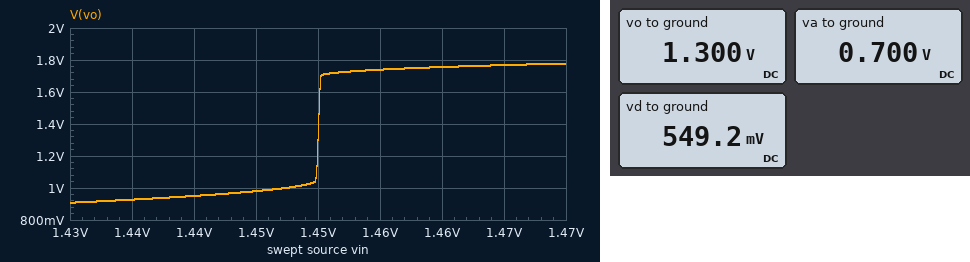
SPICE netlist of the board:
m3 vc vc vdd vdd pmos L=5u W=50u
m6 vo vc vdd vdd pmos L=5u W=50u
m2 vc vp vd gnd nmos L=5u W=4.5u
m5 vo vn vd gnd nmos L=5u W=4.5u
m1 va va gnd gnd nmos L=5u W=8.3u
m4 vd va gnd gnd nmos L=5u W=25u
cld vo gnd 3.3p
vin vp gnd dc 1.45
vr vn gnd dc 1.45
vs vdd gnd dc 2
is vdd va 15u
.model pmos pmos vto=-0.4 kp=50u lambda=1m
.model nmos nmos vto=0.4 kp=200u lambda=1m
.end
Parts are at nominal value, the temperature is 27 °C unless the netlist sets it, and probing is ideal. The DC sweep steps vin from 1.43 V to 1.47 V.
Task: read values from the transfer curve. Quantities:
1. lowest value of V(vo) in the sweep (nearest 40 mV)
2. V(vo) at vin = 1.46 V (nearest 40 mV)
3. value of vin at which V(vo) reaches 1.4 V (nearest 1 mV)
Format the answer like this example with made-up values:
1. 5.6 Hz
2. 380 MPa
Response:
1. 920 mV
2. 1.76 V
3. 1.450 V
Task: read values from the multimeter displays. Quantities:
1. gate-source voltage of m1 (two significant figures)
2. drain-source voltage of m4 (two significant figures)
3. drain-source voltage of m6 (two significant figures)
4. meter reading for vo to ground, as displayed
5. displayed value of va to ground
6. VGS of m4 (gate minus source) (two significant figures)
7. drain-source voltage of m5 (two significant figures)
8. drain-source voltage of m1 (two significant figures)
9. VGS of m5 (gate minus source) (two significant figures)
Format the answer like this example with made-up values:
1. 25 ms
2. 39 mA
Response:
1. 700 mV
2. 550 mV
3. -700 mV
4. 1.300 V
5. 0.700 V
6. 700 mV
7. 750 mV
8. 700 mV
9. 900 mV
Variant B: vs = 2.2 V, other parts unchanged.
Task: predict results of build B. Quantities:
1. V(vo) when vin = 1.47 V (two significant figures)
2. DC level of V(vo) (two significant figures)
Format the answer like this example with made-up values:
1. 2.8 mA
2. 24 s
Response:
1. 2.0 V
2. 1.5 V
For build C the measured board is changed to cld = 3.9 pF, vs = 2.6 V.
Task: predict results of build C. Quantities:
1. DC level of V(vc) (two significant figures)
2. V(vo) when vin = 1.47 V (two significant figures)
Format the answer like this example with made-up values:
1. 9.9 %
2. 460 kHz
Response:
1. 1.9 V
2. 2.4 V
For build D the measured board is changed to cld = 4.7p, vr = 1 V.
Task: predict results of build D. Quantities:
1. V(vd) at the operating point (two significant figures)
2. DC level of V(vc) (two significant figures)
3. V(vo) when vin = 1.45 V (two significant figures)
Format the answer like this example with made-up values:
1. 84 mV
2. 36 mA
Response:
1. 380 mV
2. 1.2 V
3. 2.0 V
